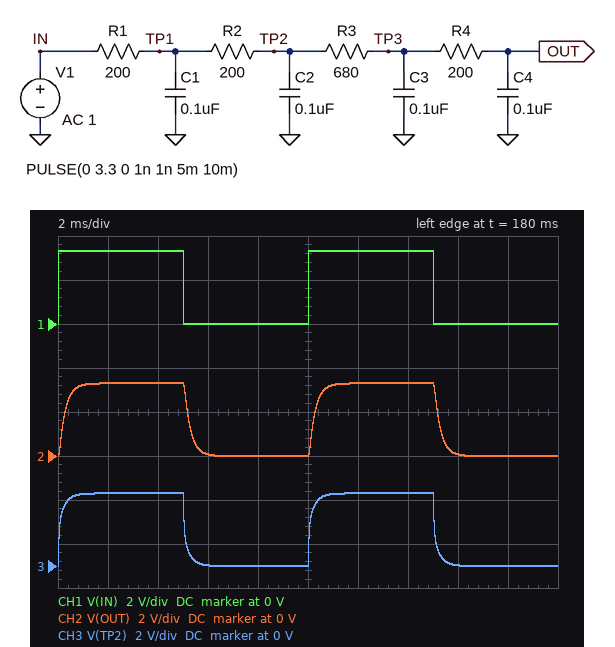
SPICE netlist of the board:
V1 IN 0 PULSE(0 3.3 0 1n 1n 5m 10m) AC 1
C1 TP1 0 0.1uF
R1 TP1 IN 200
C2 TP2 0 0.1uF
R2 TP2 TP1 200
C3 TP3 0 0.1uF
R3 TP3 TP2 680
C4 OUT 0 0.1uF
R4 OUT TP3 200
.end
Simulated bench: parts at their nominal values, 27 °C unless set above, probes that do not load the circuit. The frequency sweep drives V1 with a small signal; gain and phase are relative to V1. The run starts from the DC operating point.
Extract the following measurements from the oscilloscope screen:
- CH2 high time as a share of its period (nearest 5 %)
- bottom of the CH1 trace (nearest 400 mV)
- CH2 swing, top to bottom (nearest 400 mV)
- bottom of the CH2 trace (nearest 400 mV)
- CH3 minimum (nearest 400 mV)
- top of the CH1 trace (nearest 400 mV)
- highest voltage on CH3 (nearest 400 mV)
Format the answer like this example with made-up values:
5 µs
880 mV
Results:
50 %
0 V
3.2 V
0 V
0 V
3.2 V
3.2 V
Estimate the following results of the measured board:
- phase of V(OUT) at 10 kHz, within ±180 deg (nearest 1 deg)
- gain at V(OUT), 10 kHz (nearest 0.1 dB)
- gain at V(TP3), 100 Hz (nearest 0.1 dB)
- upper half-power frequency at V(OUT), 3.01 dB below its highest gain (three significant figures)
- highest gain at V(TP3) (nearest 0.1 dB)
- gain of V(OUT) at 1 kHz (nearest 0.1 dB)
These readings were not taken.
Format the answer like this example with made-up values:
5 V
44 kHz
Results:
155 deg
-33.1 dB
-0.1 dB
632 Hz
0 dB
-5.5 dB
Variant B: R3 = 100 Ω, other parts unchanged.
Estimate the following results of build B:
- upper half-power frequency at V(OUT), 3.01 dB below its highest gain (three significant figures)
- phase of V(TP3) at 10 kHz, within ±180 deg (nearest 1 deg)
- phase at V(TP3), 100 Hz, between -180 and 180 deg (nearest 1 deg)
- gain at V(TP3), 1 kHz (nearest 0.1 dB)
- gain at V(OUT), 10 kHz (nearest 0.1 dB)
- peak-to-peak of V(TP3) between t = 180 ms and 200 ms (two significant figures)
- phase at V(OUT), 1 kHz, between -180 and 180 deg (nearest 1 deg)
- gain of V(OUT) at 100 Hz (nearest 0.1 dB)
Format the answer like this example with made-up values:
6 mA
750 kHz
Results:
1.04 kHz
-120 deg
-6 deg
-2.8 dB
-24.1 dB
3.3 V
-54 deg
0 dB
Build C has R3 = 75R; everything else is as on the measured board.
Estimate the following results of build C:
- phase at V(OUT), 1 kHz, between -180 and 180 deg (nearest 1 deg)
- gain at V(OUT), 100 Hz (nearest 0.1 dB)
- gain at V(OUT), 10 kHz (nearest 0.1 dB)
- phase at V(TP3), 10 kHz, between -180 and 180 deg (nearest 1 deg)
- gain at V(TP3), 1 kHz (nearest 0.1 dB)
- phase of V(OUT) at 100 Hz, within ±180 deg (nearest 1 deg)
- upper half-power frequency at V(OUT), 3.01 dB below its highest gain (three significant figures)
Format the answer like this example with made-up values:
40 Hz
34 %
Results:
-53 deg
0 dB
-23.6 dB
-116 deg
-2.7 dB
-6 deg
1.06 kHz
